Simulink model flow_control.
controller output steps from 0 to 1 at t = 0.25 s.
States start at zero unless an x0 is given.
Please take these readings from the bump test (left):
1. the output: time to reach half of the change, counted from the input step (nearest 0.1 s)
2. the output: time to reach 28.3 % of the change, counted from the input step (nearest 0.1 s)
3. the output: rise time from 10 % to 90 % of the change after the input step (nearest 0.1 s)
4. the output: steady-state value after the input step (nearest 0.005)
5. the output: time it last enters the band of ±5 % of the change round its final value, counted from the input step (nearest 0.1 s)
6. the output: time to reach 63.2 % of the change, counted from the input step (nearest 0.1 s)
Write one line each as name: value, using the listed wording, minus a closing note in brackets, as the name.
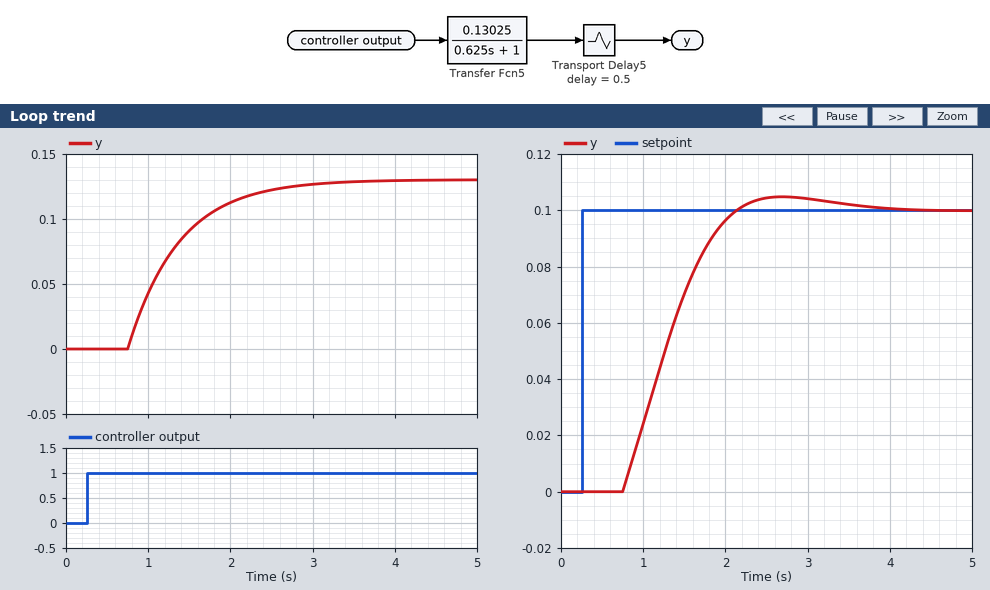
the output: time to reach half of the change, counted from the input step: 0.9 s
the output: time to reach 28.3 % of the change, counted from the input step: 0.7 s
the output: rise time from 10 % to 90 % of the change after the input step: 1.4 s
the output: steady-state value after the input step: 0.130
the output: time it last enters the band of ±5 % of the change round its final value, counted from the input step: 2.4 s
the output: time to reach 63.2 % of the change, counted from the input step: 1.1 s
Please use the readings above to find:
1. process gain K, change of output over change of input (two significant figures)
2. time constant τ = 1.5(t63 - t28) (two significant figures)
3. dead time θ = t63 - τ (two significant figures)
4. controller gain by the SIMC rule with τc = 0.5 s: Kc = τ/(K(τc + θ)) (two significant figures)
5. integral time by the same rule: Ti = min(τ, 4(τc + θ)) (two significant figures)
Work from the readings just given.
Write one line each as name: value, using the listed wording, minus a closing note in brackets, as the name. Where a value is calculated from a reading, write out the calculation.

process gain K, change of output over change of input: (0.13 - 0) / 1 = 0.13
time constant τ = 1.5(t63 - t28): 1.5 × (1.1 - 0.7) = 0.60 s
dead time θ = t63 - τ: 1.1 - 0.6 = 0.50 s
controller gain by the SIMC rule with τc = 0.5 s: Kc = τ/(K(τc + θ)): 0.6 / (0.13 × (0.5 + 0.5)) = 4.6
integral time by the same rule: Ti = min(τ, 4(τc + θ)): min(0.6, 4 × (0.5 + 0.5)) = 0.60 s
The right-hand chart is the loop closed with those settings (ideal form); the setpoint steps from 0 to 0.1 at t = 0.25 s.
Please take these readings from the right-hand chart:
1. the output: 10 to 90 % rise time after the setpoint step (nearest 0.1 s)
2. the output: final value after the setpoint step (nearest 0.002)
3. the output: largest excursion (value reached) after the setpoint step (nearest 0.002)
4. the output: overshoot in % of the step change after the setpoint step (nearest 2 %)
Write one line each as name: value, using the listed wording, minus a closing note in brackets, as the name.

the output: 10 to 90 % rise time after the setpoint step: 1.0 s
the output: final value after the setpoint step: 0.100
the output: largest excursion (value reached) after the setpoint step: 0.104
the output: overshoot in % of the step change after the setpoint step: 4 %
